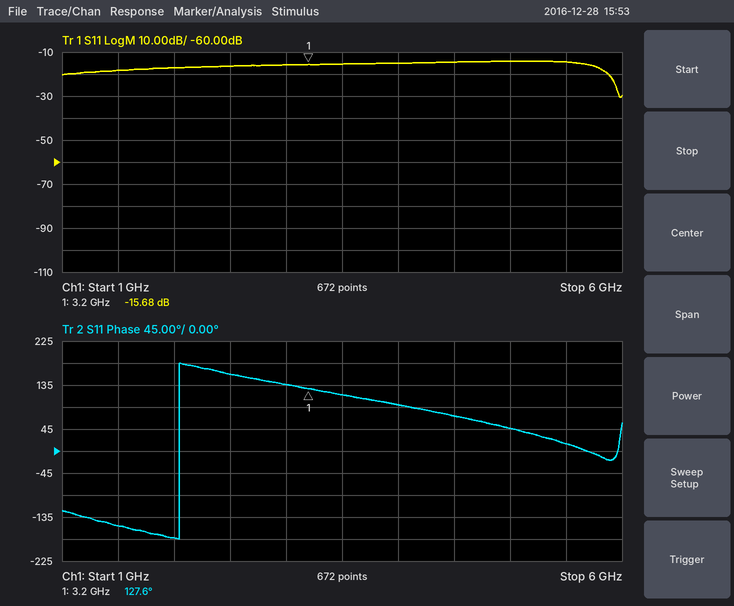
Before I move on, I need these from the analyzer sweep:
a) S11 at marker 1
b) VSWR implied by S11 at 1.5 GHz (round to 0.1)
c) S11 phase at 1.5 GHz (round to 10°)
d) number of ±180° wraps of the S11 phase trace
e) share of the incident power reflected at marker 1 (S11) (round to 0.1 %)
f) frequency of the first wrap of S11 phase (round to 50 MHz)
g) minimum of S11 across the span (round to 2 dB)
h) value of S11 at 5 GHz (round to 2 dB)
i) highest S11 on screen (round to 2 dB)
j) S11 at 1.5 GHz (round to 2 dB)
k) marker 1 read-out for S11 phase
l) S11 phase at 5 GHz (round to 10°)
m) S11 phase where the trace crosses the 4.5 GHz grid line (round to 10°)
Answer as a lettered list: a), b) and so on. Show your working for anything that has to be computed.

a) -15.68 dB
b) |Γ| = 10^(-18/20) = 0.1259; VSWR = (1 + 0.1259)/(1 − 0.1259) ≈ 1.3
c) -150°
d) 1
e) 10^(-15.68/10) ≈ 2.7 %
f) 2.05 GHz
g) -30 dB
h) -14 dB
i) -14 dB
j) -18 dB
k) 127.6°
l) 50°
m) 70°
